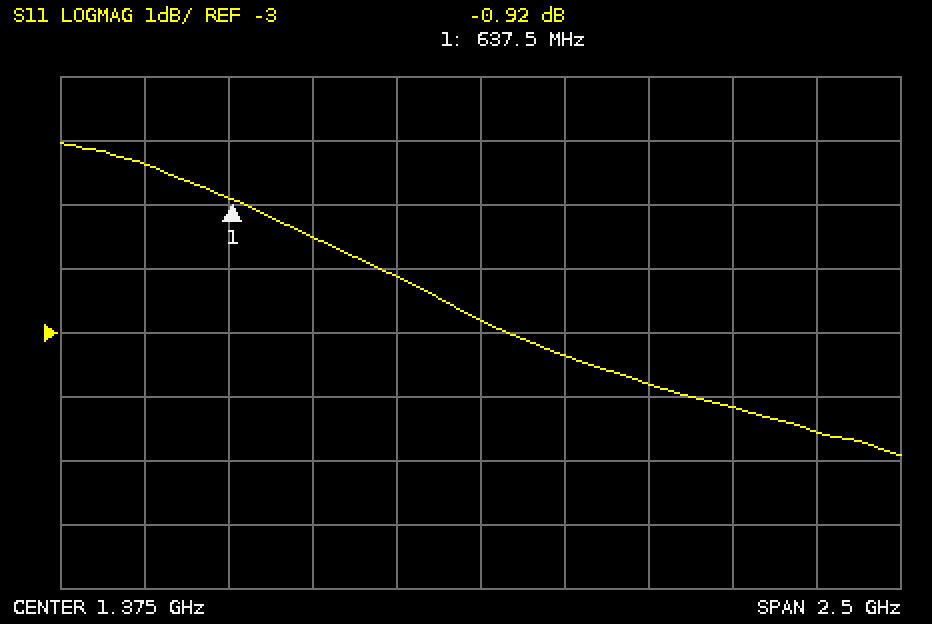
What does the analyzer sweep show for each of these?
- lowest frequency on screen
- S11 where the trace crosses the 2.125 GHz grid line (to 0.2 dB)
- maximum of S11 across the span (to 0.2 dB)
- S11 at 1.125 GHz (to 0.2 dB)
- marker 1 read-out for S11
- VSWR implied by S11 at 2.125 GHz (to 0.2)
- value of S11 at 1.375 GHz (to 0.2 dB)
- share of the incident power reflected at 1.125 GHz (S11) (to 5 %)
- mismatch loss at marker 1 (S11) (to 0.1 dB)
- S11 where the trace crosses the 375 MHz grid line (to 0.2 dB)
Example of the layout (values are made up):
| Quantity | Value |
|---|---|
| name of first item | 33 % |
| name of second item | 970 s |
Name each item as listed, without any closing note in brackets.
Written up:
| Quantity | Value |
|---|---|
| lowest frequency on screen | 125 MHz |
| S11 where the trace crosses the 2.125 GHz grid line | -4.2 dB |
| maximum of S11 across the span | 0.0 dB |
| S11 at 1.125 GHz | -2.2 dB |
| marker 1 read-out for S11 | -0.92 dB |
| VSWR implied by S11 at 2.125 GHz | 4.2 |
| value of S11 at 1.375 GHz | -2.8 dB |
| share of the incident power reflected at 1.125 GHz (S11) | 60 % |
| mismatch loss at marker 1 (S11) | 7.2 dB |
| S11 where the trace crosses the 375 MHz grid line | -0.4 dB |
